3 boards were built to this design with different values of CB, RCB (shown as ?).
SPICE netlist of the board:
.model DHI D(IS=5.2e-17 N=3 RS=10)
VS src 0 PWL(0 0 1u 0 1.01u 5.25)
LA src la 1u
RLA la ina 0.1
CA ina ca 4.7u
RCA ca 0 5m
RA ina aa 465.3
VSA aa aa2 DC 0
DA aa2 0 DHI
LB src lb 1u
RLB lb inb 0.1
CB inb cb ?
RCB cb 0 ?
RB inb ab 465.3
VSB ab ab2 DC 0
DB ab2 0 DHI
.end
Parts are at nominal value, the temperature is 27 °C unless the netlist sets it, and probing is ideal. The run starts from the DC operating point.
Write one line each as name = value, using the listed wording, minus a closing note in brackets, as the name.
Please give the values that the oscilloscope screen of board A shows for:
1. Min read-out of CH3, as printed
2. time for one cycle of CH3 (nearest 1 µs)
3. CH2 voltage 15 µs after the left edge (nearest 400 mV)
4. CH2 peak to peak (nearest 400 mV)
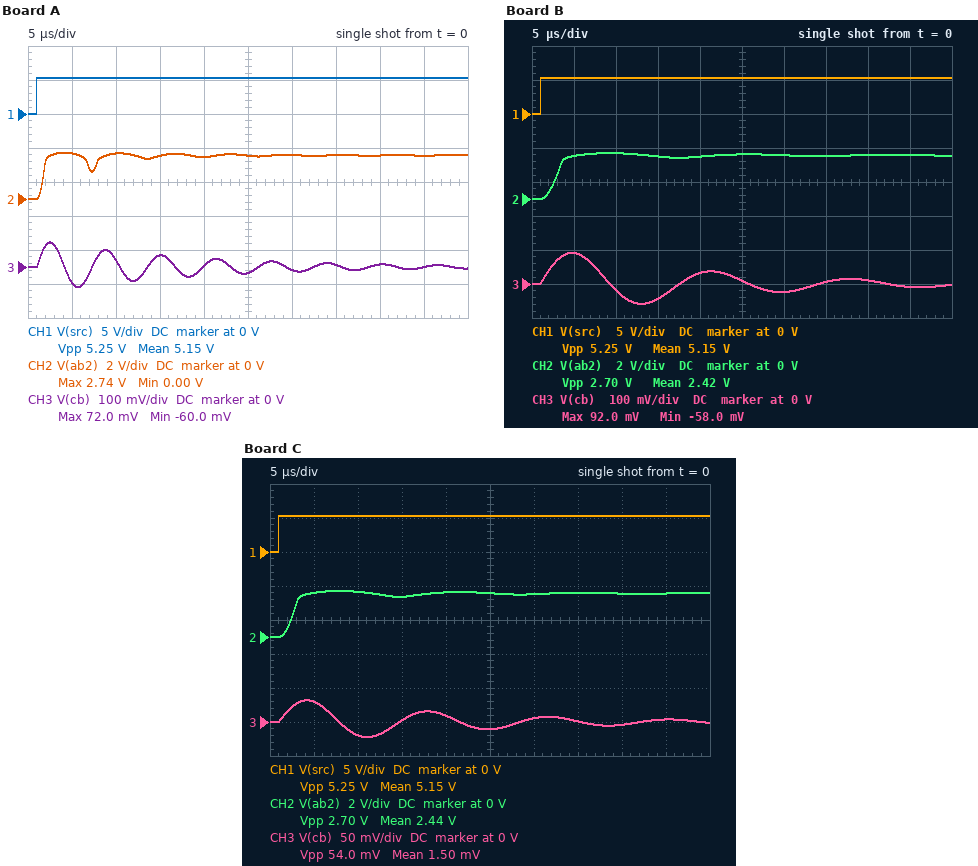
Min read-out of CH3, as printed = -60.0 mV
time for one cycle of CH3 = 6 µs
CH2 voltage 15 µs after the left edge = 2.4 V
CH2 peak to peak = 2.8 V
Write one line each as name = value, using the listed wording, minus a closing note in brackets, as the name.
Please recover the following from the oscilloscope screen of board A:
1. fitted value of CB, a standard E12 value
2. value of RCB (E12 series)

fitted value of CB, a standard E12 value = 1 µF
value of RCB = 0.015 Ω
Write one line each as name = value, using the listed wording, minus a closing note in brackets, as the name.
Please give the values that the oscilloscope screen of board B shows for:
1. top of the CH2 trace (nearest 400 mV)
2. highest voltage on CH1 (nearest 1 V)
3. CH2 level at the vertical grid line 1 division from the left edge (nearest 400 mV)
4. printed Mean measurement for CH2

top of the CH2 trace = 2.8 V
highest voltage on CH1 = 5 V
CH2 level at the vertical grid line 1 division from the left edge = 2.4 V
printed Mean measurement for CH2 = 2.42 V
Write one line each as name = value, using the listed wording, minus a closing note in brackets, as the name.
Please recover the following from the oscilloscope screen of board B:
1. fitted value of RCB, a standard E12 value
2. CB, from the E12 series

fitted value of RCB, a standard E12 value = 8.2 mΩ
CB, from the E12 series = 6.8 µF
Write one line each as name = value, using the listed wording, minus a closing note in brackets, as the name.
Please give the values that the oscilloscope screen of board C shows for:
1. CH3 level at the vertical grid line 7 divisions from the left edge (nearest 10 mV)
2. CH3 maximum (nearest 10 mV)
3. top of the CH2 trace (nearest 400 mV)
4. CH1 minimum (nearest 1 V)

CH3 level at the vertical grid line 7 divisions from the left edge = 0 V
CH3 maximum = 30 mV
top of the CH2 trace = 2.8 V
CH1 minimum = 0 V
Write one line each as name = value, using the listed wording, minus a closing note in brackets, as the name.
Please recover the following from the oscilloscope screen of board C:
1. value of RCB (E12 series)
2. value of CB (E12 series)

value of RCB = 3.3 mΩ
value of CB = 4.7 µF
